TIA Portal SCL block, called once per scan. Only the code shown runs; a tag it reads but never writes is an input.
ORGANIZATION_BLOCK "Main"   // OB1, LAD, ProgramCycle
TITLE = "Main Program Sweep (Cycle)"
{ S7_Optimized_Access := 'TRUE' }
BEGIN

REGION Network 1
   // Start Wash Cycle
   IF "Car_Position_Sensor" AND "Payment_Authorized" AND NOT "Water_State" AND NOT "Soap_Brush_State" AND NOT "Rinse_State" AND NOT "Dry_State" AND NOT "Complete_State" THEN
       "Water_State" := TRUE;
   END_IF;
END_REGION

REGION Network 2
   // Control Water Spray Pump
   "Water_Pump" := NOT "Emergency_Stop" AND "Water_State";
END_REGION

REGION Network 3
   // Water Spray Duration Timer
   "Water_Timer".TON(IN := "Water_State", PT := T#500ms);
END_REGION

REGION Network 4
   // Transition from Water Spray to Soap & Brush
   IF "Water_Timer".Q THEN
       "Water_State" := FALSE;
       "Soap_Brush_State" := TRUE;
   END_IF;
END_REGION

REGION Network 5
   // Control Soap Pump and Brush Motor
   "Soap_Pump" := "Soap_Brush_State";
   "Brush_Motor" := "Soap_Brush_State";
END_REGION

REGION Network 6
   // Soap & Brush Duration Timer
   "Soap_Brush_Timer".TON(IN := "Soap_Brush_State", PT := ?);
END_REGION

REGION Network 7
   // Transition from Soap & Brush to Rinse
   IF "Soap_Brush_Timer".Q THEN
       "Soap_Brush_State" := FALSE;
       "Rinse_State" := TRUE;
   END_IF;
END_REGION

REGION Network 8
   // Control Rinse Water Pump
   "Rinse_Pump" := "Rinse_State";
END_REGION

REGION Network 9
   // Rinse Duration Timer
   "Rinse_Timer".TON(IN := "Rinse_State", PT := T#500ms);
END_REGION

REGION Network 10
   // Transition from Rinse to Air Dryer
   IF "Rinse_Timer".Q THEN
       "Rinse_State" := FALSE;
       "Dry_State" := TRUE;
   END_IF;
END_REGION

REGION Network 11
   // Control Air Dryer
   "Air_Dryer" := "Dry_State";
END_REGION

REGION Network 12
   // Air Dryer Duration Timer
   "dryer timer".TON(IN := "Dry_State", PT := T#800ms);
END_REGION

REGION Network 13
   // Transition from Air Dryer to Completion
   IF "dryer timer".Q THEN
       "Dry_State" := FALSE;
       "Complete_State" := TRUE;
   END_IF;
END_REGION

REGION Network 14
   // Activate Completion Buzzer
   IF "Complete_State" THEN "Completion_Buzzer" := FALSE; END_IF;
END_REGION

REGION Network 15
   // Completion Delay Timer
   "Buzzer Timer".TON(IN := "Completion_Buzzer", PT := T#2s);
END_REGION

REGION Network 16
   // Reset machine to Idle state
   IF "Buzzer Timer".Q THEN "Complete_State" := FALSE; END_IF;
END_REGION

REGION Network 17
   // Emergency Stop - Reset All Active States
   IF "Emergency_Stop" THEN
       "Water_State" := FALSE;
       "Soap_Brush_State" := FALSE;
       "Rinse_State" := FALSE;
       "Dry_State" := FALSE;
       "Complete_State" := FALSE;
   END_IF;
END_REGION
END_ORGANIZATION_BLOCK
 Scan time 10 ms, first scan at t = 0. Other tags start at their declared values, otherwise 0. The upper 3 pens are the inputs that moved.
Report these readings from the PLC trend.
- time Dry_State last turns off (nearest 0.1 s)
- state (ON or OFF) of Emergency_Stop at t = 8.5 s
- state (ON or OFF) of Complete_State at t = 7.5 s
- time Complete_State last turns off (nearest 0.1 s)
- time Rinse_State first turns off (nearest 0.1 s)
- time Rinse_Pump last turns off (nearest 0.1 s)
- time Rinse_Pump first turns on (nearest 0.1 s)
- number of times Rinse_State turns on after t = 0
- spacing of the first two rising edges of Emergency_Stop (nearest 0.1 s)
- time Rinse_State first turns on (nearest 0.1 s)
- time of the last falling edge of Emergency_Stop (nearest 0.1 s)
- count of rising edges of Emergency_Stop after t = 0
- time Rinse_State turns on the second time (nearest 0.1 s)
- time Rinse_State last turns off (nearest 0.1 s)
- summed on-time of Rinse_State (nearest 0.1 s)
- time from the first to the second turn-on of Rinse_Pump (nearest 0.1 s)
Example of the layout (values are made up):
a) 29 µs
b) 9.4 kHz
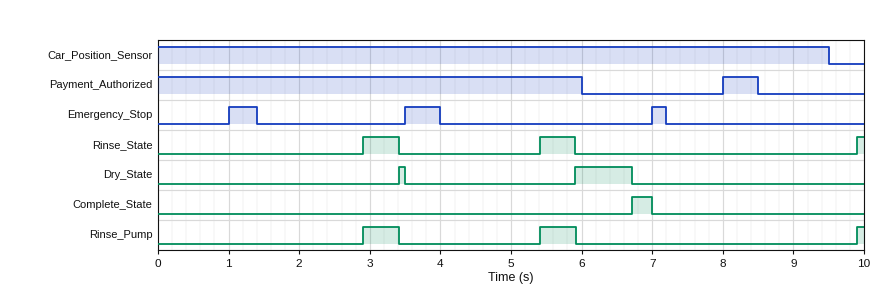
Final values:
a) 6.7 s
b) OFF
c) OFF
d) 7.0 s
e) 3.4 s
f) 5.9 s
g) 2.9 s
h) 3
i) 2.5 s
j) 2.9 s
k) 7.2 s
l) 3
m) 5.4 s
n) 5.9 s
o) 1.1 s
p) 2.5 s
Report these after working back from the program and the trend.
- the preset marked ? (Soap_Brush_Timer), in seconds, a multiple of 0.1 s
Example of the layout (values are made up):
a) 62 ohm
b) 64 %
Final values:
a) 1.4 s
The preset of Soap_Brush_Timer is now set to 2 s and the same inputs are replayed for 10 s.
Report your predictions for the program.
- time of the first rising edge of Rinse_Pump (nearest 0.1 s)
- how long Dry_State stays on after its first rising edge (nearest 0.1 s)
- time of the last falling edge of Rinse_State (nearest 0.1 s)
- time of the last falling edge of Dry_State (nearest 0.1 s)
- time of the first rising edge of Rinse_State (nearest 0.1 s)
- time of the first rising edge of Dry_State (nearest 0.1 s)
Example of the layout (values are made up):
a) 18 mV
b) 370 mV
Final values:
a) 6.0 s
b) 0.5 s
c) 6.5 s
d) 7.0 s
e) 6.0 s
f) 6.5 s
